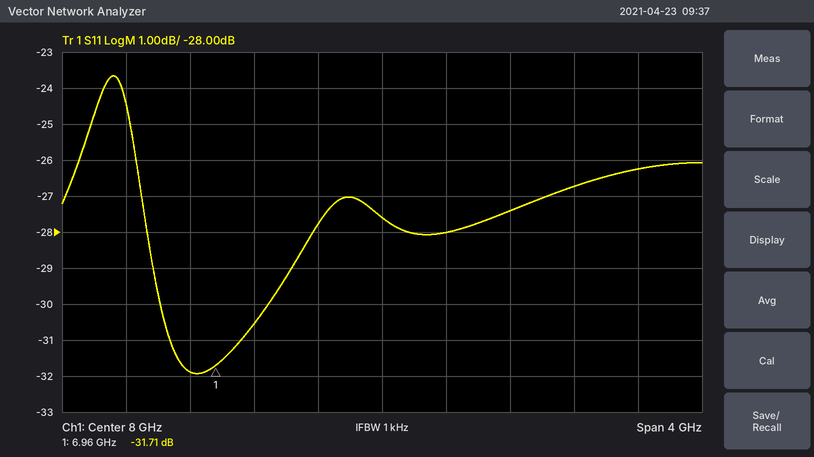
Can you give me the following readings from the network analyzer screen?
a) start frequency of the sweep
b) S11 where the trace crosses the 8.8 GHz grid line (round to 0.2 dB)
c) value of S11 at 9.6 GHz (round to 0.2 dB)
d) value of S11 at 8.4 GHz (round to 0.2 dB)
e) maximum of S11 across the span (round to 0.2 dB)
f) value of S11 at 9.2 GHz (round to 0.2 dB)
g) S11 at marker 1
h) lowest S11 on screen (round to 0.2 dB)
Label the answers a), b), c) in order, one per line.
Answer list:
a) 6 GHz
b) -27.4 dB
c) -26.2 dB
d) -28.0 dB
e) -23.6 dB
f) -26.8 dB
g) -31.71 dB
h) -32.0 dB
